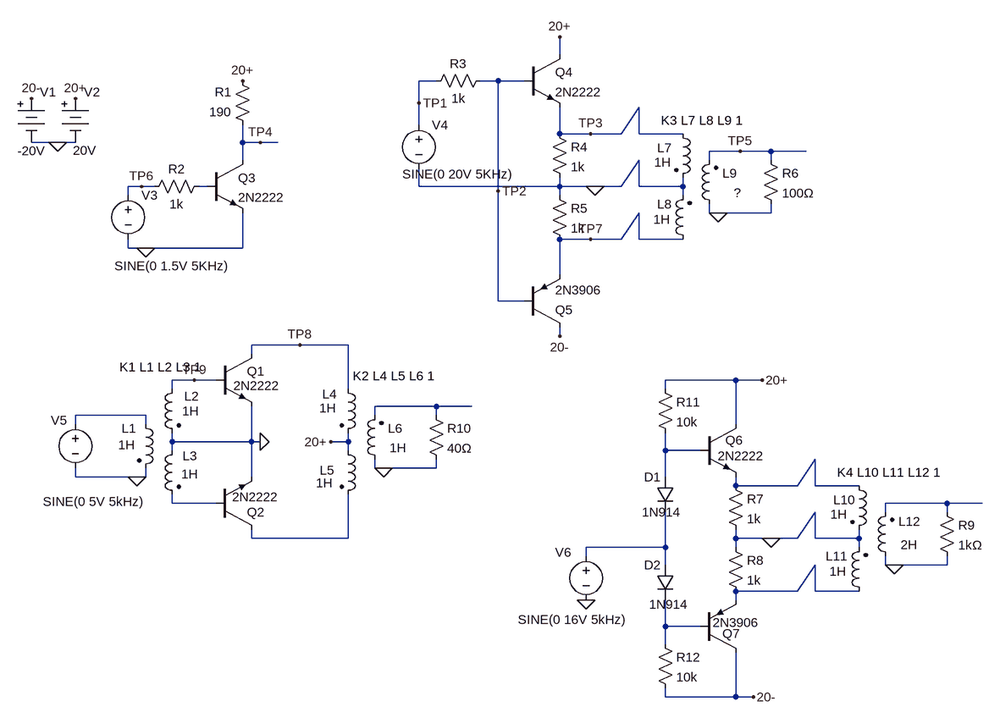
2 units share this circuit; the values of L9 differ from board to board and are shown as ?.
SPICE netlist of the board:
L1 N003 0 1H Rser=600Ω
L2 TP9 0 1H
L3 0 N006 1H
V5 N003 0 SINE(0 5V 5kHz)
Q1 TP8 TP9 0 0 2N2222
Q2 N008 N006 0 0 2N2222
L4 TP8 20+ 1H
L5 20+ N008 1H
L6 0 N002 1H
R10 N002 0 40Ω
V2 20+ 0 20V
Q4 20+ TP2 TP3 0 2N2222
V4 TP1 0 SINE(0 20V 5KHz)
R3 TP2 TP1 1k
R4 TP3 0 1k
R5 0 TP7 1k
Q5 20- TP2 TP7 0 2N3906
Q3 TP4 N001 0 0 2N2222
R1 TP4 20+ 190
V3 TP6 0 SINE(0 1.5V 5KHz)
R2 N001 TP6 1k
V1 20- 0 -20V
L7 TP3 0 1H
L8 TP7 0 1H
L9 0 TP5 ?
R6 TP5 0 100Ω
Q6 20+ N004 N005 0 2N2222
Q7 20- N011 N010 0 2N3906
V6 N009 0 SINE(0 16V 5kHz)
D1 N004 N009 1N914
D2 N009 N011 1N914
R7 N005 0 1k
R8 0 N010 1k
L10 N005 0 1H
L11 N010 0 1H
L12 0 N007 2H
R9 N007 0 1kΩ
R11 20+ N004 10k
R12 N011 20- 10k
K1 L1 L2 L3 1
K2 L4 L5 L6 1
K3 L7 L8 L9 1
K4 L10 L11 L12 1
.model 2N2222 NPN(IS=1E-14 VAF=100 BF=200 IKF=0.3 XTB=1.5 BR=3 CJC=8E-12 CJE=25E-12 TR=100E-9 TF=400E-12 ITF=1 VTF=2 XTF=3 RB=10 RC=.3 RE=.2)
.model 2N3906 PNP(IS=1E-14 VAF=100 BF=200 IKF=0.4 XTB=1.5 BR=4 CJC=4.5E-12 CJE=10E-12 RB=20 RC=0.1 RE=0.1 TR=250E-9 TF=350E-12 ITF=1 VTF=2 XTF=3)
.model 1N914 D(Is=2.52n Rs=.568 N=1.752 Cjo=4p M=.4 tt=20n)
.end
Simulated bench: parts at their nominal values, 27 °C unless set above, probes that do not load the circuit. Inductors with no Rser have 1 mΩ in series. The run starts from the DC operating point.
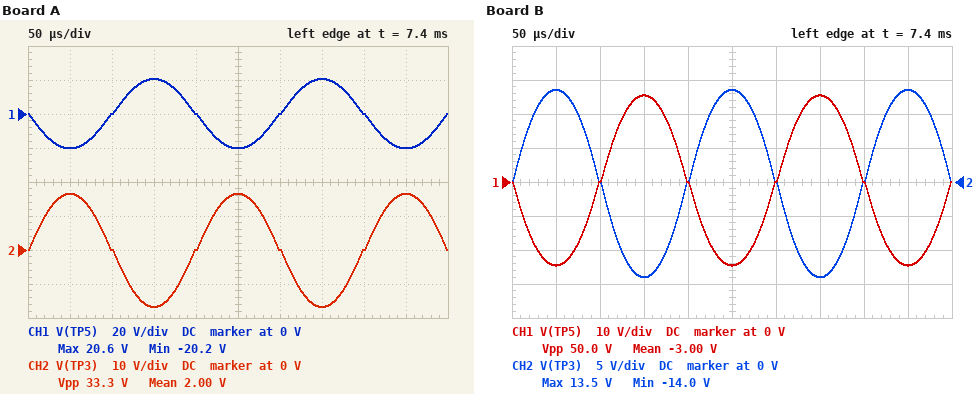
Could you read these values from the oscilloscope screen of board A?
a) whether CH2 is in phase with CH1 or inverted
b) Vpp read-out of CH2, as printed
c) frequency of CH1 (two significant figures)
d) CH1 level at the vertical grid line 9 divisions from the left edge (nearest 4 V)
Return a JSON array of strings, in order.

["inverted", "33.3 V", "5.0 kHz", "-20 V"]
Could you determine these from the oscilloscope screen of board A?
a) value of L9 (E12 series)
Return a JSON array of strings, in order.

["1.5 H"]
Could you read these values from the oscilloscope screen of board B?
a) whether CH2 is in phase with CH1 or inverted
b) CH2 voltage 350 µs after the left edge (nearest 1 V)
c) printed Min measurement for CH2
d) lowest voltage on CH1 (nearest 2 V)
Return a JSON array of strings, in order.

["inverted", "-14 V", "-14.0 V", "-24 V"]
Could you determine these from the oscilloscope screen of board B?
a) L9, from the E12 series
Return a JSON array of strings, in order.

["3.3 H"]
